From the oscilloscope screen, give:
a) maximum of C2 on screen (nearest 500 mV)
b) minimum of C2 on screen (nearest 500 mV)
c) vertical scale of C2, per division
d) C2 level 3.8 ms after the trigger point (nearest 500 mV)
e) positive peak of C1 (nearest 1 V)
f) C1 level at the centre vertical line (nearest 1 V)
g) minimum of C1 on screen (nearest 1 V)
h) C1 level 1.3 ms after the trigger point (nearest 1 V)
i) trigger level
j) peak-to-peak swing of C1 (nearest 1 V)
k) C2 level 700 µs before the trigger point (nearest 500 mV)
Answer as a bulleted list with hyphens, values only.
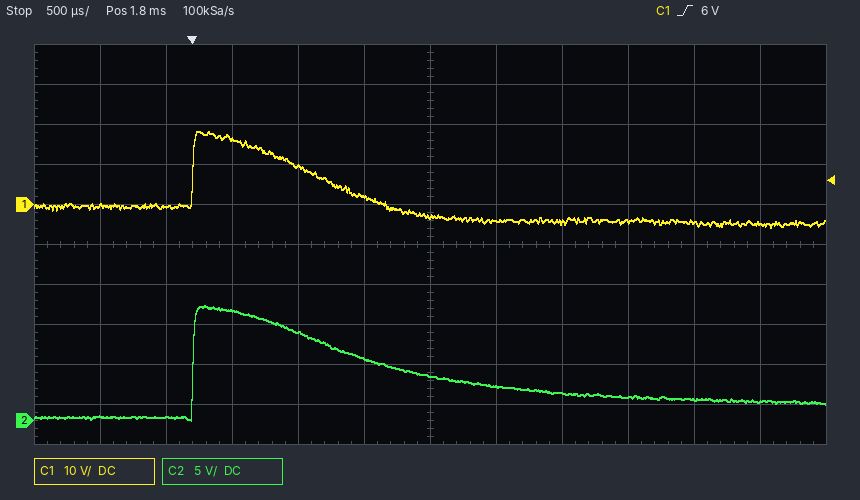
- 14.5 V
- 0.0 V
- 5 V
- 2.5 V
- 18 V
- -3 V
- -6 V
- 2 V
- 6 V
- 24 V
- 500 mV
